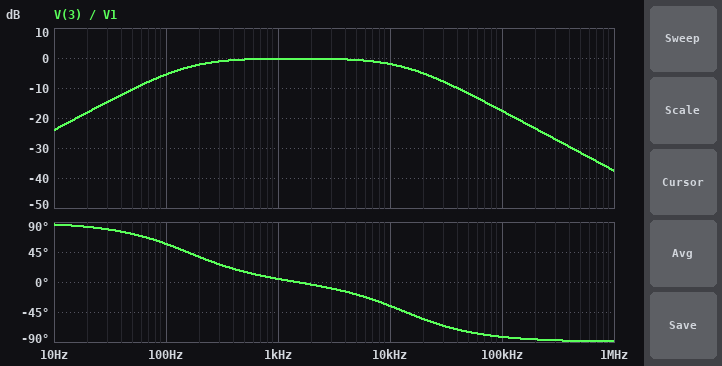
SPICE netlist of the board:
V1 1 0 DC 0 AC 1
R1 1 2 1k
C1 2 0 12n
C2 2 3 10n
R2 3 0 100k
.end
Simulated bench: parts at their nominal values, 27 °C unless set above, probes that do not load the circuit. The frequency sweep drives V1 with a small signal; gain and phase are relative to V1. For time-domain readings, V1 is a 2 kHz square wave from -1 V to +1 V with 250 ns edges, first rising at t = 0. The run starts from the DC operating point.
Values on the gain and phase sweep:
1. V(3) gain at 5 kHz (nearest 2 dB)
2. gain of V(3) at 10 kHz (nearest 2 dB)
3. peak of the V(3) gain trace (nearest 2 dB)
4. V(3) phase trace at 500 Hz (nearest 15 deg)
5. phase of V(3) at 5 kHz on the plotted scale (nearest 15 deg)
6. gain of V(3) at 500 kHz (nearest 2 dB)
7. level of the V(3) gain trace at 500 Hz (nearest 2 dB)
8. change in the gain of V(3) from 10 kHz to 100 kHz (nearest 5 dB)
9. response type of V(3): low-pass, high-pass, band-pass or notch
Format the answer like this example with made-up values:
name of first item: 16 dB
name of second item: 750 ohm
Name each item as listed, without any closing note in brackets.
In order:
V(3) gain at 5 kHz: 0 dB
gain of V(3) at 10 kHz: -2 dB
peak of the V(3) gain trace: 0 dB
V(3) phase trace at 500 Hz: 15 deg
phase of V(3) at 5 kHz on the plotted scale: -15 deg
gain of V(3) at 500 kHz: -32 dB
level of the V(3) gain trace at 500 Hz: 0 dB
change in the gain of V(3) from 10 kHz to 100 kHz: -15 dB
response type of V(3): low-pass, high-pass, band-pass or notch: band-pass
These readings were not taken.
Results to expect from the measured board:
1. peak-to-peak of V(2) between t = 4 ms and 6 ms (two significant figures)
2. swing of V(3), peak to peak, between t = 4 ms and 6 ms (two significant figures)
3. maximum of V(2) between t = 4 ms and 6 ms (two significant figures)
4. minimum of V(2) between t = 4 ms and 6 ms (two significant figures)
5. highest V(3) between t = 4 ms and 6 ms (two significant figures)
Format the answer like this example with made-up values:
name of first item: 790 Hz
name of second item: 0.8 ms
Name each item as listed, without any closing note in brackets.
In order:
peak-to-peak of V(2) between t = 4 ms and 6 ms: 2.0 V
swing of V(3), peak to peak, between t = 4 ms and 6 ms: 2.1 V
maximum of V(2) between t = 4 ms and 6 ms: 990 mV
minimum of V(2) between t = 4 ms and 6 ms: -990 mV
highest V(3) between t = 4 ms and 6 ms: 1.1 V
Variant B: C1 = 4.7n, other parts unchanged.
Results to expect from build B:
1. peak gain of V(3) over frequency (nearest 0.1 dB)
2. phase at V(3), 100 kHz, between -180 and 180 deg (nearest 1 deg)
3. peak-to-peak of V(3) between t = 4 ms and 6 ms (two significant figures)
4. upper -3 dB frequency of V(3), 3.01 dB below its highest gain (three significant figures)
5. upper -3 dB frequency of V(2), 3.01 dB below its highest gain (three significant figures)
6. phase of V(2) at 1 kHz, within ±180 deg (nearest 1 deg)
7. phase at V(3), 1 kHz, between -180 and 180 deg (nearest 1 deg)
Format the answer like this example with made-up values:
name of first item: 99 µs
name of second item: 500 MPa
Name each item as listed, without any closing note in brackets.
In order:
peak gain of V(3) over frequency: -0.1 dB
phase at V(3), 100 kHz, between -180 and 180 deg: -71 deg
peak-to-peak of V(3) between t = 4 ms and 6 ms: 2.2 V
upper -3 dB frequency of V(3), 3.01 dB below its highest gain: 34.5 kHz
upper -3 dB frequency of V(2), 3.01 dB below its highest gain: 33.5 kHz
phase of V(2) at 1 kHz, within ±180 deg: -2 deg
phase at V(3), 1 kHz, between -180 and 180 deg: 7 deg
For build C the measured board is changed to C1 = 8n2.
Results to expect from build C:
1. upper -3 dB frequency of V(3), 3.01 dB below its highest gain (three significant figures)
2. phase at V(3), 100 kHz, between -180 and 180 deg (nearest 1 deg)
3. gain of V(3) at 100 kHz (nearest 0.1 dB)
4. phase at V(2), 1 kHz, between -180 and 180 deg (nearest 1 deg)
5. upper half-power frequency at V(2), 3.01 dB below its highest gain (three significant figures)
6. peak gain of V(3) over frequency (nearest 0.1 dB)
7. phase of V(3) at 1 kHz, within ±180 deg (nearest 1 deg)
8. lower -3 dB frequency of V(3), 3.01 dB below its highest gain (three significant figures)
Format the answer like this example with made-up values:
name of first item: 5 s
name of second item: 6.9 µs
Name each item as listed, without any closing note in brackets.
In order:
upper -3 dB frequency of V(3), 3.01 dB below its highest gain: 19.9 kHz
phase at V(3), 100 kHz, between -180 and 180 deg: -79 deg
gain of V(3) at 100 kHz: -14.4 dB
phase at V(2), 1 kHz, between -180 and 180 deg: -3 deg
upper half-power frequency at V(2), 3.01 dB below its highest gain: 19.2 kHz
peak gain of V(3) over frequency: -0.2 dB
phase of V(3) at 1 kHz, within ±180 deg: 6 deg
lower -3 dB frequency of V(3), 3.01 dB below its highest gain: 155 Hz
